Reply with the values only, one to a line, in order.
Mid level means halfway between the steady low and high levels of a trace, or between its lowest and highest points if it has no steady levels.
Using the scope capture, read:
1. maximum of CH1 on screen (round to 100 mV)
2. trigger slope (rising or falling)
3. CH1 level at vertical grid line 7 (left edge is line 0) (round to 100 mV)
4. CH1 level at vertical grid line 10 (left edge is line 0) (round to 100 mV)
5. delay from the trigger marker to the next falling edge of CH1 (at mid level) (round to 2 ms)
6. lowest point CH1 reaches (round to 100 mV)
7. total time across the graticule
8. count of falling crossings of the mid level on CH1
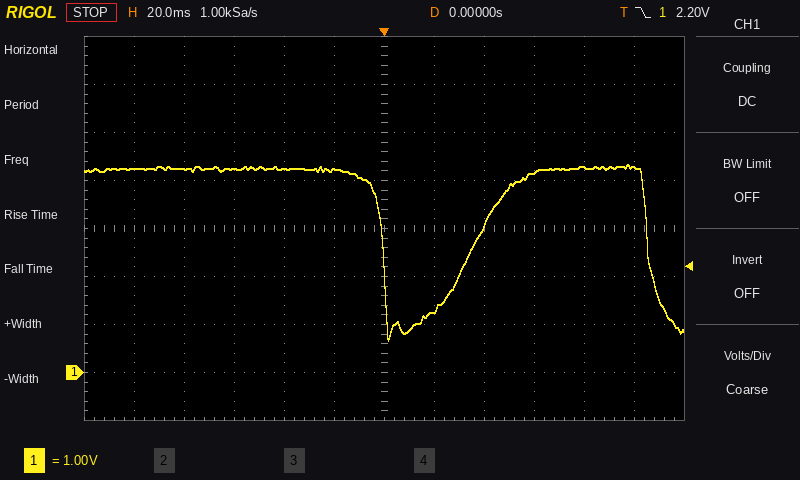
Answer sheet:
4.3 V
falling
1.3 V
4.3 V
106 ms
700 mV
240 ms
2
